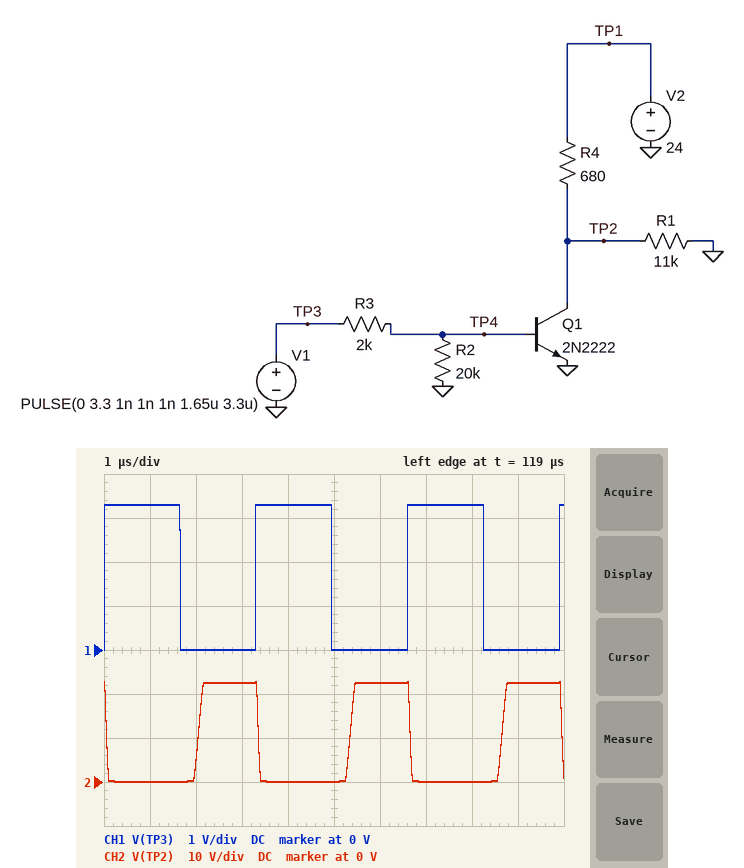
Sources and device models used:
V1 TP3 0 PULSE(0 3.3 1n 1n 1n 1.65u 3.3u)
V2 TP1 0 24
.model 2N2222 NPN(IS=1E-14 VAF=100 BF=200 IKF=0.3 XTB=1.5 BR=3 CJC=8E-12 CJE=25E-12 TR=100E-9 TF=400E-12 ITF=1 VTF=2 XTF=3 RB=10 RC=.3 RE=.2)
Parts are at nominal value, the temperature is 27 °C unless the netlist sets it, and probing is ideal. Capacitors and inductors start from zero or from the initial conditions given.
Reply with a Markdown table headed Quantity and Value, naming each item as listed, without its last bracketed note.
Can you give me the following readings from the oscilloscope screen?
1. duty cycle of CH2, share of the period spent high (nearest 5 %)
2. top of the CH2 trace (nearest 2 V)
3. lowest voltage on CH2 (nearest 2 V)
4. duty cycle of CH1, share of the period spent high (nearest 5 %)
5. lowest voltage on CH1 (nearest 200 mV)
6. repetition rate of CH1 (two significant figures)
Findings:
| Quantity | Value |
|---|---|
| duty cycle of CH2, share of the period spent high | 40 % |
| top of the CH2 trace | 22 V |
| lowest voltage on CH2 | 0 V |
| duty cycle of CH1, share of the period spent high | 50 % |
| lowest voltage on CH1 | 0 V |
| repetition rate of CH1 | 300 kHz |
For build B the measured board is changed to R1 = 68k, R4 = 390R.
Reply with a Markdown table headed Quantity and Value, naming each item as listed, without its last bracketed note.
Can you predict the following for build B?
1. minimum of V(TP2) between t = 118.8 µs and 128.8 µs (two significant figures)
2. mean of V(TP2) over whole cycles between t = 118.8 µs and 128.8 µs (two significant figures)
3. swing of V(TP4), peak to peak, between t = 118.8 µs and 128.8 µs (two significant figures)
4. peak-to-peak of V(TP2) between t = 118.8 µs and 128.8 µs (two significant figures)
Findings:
| Quantity | Value |
|---|---|
| minimum of V(TP2) between t = 118.8 µs and 128.8 µs | 120 mV |
| mean of V(TP2) over whole cycles between t = 118.8 µs and 128.8 µs | 10 V |
| swing of V(TP4), peak to peak, between t = 118.8 µs and 128.8 µs | 790 mV |
| peak-to-peak of V(TP2) between t = 118.8 µs and 128.8 µs | 24 V |
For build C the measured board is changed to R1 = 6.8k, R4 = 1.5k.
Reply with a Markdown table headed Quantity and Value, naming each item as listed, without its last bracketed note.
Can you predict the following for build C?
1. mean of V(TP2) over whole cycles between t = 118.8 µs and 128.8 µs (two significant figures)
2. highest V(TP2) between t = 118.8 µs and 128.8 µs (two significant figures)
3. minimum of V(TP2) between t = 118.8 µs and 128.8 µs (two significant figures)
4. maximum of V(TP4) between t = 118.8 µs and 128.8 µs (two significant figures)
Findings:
| Quantity | Value |
|---|---|
| mean of V(TP2) over whole cycles between t = 118.8 µs and 128.8 µs | 7.3 V |
| highest V(TP2) between t = 118.8 µs and 128.8 µs | 20 V |
| minimum of V(TP2) between t = 118.8 µs and 128.8 µs | 54 mV |
| maximum of V(TP4) between t = 118.8 µs and 128.8 µs | 750 mV |
